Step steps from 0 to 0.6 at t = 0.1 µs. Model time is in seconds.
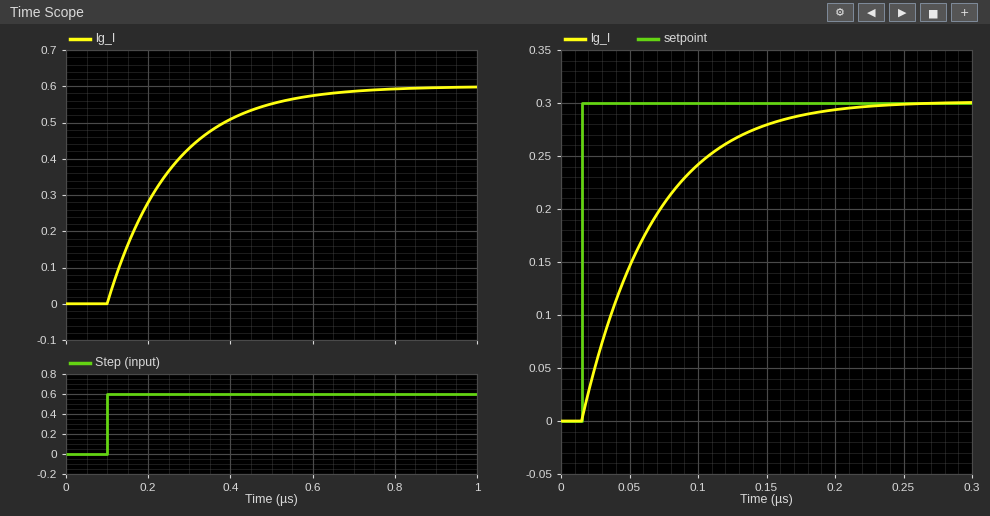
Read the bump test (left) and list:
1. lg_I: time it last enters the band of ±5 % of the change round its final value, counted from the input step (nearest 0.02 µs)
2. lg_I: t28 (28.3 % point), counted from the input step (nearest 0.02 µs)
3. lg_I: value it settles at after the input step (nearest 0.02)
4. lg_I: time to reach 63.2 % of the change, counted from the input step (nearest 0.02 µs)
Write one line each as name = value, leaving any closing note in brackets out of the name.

lg_I: time it last enters the band of ±5 % of the change round its final value, counted from the input step = 0.48 µs
lg_I: t28 (28.3 % point), counted from the input step = 0.06 µs
lg_I: value it settles at after the input step = 0.60
lg_I: time to reach 63.2 % of the change, counted from the input step = 0.16 µs
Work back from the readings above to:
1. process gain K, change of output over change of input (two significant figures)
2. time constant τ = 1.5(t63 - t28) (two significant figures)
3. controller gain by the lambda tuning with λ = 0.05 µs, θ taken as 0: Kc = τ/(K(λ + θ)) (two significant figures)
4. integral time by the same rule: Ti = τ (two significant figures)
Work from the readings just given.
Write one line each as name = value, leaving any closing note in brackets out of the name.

process gain K, change of output over change of input = 1.0
time constant τ = 1.5(t63 - t28) = 0.15 µs
controller gain by the lambda tuning with λ = 0.05 µs, θ taken as 0: Kc = τ/(K(λ + θ)) = 3.0
integral time by the same rule: Ti = τ = 0.15 µs
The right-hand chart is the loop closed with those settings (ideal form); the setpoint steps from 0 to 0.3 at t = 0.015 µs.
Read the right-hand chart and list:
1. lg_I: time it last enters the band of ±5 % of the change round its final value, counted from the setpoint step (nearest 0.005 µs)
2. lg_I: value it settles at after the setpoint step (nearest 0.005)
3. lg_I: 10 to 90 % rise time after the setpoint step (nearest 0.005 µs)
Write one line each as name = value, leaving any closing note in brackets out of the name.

lg_I: time it last enters the band of ±5 % of the change round its final value, counted from the setpoint step = 0.150 µs
lg_I: value it settles at after the setpoint step = 0.300
lg_I: 10 to 90 % rise time after the setpoint step = 0.110 µs
